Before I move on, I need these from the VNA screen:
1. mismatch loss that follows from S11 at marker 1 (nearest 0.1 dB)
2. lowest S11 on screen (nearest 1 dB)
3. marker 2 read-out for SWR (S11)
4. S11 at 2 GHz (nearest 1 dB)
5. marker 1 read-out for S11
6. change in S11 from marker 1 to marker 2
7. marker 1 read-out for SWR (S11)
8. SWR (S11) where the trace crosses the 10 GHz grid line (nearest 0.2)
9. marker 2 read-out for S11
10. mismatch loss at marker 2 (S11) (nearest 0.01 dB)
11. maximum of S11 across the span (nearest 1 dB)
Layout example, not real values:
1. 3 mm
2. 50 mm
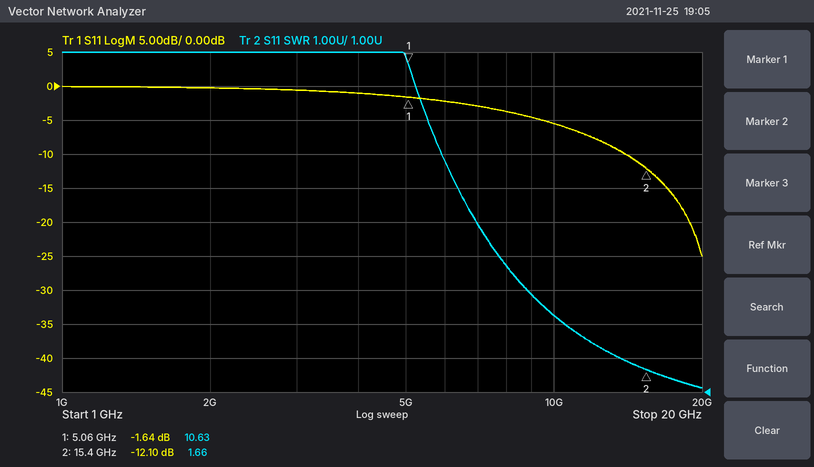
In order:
1. 5.0 dB
2. -25 dB
3. 1.66
4. 0 dB
5. -1.64 dB
6. -10.46 dB
7. 10.63
8. 3.2
9. -12.10 dB
10. 0.28 dB
11. 0 dB
